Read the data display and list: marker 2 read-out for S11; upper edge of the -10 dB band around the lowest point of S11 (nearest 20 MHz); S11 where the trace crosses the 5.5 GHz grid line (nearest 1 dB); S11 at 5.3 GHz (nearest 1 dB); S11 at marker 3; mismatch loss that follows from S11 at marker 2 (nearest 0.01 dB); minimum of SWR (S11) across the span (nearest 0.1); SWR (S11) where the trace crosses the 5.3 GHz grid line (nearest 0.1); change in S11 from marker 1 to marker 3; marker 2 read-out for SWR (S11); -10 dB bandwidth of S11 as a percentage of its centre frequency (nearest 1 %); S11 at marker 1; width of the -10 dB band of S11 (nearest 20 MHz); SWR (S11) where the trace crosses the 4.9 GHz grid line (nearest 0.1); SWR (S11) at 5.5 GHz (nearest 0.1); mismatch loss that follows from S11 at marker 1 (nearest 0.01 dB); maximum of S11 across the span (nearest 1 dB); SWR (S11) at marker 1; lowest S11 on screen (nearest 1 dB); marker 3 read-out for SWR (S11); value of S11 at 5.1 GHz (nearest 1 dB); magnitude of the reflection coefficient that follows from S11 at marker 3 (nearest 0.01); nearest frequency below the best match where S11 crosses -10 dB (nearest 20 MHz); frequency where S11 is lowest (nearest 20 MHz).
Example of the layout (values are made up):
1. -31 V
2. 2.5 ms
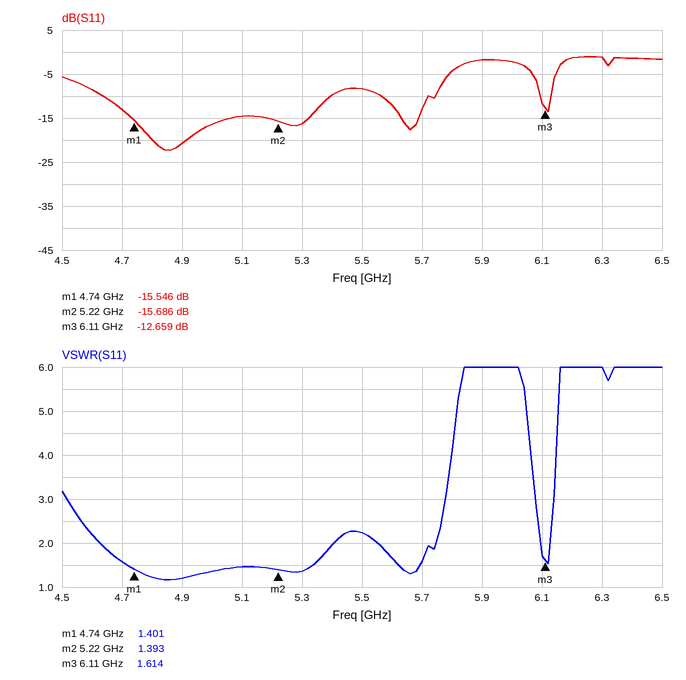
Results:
1. -15.686 dB
2. 5.40 GHz
3. -8 dB
4. -16 dB
5. -12.659 dB
6. 0.12 dB
7. 1.2
8. 1.4
9. 2.887 dB
10. 1.393
11. 15 %
12. -15.546 dB
13. 760 MHz
14. 1.2
15. 2.2
16. 0.12 dB
17. -1 dB
18. 1.401
19. -22 dB
20. 1.614
21. -15 dB
22. 0.23
23. 4.64 GHz
24. 4.86 GHz
